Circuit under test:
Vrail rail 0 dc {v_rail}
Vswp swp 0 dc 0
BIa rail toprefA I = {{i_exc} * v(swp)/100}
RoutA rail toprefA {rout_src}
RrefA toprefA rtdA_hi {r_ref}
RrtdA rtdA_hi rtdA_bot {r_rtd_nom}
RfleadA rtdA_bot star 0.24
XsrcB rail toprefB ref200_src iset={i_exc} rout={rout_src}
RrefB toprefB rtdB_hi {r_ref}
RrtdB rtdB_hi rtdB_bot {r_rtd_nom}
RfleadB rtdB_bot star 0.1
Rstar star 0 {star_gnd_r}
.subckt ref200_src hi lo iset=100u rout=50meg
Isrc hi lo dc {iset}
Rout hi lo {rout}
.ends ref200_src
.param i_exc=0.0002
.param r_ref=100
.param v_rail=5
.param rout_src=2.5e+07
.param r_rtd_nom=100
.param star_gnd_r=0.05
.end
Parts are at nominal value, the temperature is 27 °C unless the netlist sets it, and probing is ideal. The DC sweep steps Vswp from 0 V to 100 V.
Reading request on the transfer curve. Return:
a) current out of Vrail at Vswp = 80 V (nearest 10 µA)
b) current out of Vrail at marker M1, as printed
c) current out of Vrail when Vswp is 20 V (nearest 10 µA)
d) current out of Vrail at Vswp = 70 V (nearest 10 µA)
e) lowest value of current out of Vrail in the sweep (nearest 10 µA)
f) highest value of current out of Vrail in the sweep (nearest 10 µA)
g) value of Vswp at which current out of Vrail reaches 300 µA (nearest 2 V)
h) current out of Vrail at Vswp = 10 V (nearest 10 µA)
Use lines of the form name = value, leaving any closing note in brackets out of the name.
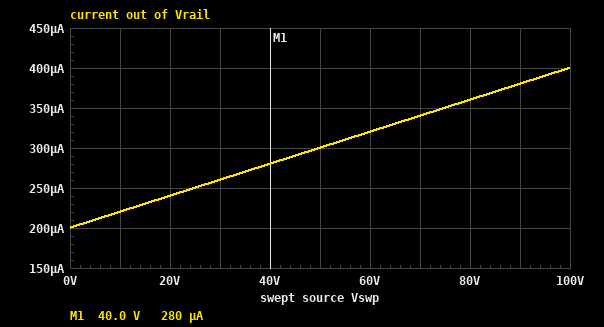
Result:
current out of Vrail at Vswp = 80 V = 360 µA
current out of Vrail at marker M1, as printed = 280 µA
current out of Vrail when Vswp is 20 V = 240 µA
current out of Vrail at Vswp = 70 V = 340 µA
lowest value of current out of Vrail in the sweep = 200 µA
highest value of current out of Vrail in the sweep = 400 µA
value of Vswp at which current out of Vrail reaches 300 µA = 50 V
current out of Vrail at Vswp = 10 V = 220 µA
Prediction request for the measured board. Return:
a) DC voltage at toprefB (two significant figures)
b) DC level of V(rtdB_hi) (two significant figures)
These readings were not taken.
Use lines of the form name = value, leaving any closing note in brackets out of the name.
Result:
DC voltage at toprefB = 40 mV
DC level of V(rtdB_hi) = 20 mV
